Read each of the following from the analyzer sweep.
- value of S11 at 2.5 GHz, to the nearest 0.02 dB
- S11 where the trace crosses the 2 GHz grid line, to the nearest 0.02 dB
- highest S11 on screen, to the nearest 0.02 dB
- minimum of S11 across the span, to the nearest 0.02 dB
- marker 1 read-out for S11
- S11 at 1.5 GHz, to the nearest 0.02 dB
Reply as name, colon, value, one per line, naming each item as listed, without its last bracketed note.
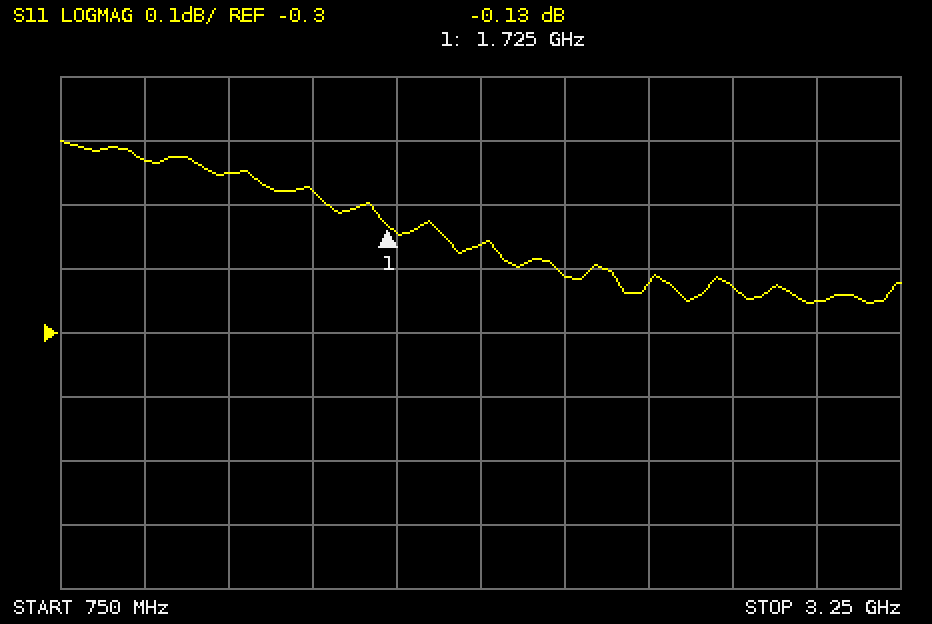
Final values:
value of S11 at 2.5 GHz, to the nearest 0.02 dB: -0.22 dB
S11 where the trace crosses the 2 GHz grid line, to the nearest 0.02 dB: -0.16 dB
highest S11 on screen, to the nearest 0.02 dB: 0.00 dB
minimum of S11 across the span, to the nearest 0.02 dB: -0.26 dB
marker 1 read-out for S11: -0.13 dB
S11 at 1.5 GHz, to the nearest 0.02 dB: -0.08 dB
